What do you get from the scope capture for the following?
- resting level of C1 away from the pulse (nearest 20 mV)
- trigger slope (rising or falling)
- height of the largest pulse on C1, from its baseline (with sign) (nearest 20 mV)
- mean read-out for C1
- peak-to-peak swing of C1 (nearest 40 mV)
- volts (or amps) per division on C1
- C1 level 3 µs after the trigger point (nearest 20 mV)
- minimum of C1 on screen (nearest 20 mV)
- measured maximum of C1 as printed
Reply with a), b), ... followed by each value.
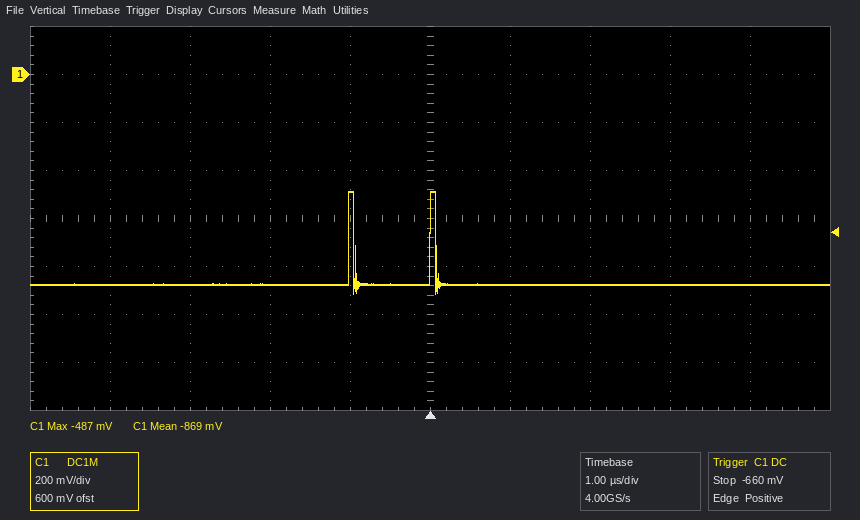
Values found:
a) -880 mV
b) rising
c) +380 mV
d) -869 mV
e) 440 mV
f) 200 mV
g) -880 mV
h) -920 mV
i) -487 mV
